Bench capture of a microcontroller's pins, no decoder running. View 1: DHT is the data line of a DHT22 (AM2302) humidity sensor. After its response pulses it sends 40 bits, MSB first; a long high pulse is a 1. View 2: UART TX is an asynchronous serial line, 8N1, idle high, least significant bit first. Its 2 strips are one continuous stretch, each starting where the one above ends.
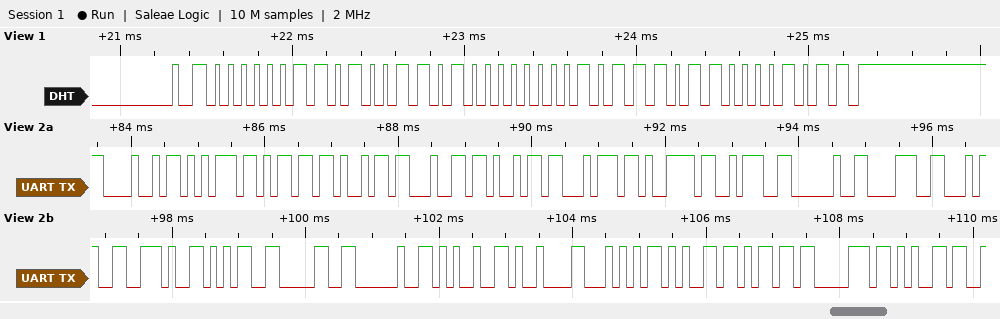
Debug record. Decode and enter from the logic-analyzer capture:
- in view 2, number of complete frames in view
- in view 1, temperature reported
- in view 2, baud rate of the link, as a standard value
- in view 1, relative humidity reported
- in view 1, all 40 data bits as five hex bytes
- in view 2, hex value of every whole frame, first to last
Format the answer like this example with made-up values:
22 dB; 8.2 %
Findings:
23; 18.7 °C; 9600 baud; 84.5 %; 03 4D 00 BB 0B; 48 75 6D 69 64 69 74 79 3A 20 38 34 2E 35 30 20 25 09 54 65 6D 70 65
